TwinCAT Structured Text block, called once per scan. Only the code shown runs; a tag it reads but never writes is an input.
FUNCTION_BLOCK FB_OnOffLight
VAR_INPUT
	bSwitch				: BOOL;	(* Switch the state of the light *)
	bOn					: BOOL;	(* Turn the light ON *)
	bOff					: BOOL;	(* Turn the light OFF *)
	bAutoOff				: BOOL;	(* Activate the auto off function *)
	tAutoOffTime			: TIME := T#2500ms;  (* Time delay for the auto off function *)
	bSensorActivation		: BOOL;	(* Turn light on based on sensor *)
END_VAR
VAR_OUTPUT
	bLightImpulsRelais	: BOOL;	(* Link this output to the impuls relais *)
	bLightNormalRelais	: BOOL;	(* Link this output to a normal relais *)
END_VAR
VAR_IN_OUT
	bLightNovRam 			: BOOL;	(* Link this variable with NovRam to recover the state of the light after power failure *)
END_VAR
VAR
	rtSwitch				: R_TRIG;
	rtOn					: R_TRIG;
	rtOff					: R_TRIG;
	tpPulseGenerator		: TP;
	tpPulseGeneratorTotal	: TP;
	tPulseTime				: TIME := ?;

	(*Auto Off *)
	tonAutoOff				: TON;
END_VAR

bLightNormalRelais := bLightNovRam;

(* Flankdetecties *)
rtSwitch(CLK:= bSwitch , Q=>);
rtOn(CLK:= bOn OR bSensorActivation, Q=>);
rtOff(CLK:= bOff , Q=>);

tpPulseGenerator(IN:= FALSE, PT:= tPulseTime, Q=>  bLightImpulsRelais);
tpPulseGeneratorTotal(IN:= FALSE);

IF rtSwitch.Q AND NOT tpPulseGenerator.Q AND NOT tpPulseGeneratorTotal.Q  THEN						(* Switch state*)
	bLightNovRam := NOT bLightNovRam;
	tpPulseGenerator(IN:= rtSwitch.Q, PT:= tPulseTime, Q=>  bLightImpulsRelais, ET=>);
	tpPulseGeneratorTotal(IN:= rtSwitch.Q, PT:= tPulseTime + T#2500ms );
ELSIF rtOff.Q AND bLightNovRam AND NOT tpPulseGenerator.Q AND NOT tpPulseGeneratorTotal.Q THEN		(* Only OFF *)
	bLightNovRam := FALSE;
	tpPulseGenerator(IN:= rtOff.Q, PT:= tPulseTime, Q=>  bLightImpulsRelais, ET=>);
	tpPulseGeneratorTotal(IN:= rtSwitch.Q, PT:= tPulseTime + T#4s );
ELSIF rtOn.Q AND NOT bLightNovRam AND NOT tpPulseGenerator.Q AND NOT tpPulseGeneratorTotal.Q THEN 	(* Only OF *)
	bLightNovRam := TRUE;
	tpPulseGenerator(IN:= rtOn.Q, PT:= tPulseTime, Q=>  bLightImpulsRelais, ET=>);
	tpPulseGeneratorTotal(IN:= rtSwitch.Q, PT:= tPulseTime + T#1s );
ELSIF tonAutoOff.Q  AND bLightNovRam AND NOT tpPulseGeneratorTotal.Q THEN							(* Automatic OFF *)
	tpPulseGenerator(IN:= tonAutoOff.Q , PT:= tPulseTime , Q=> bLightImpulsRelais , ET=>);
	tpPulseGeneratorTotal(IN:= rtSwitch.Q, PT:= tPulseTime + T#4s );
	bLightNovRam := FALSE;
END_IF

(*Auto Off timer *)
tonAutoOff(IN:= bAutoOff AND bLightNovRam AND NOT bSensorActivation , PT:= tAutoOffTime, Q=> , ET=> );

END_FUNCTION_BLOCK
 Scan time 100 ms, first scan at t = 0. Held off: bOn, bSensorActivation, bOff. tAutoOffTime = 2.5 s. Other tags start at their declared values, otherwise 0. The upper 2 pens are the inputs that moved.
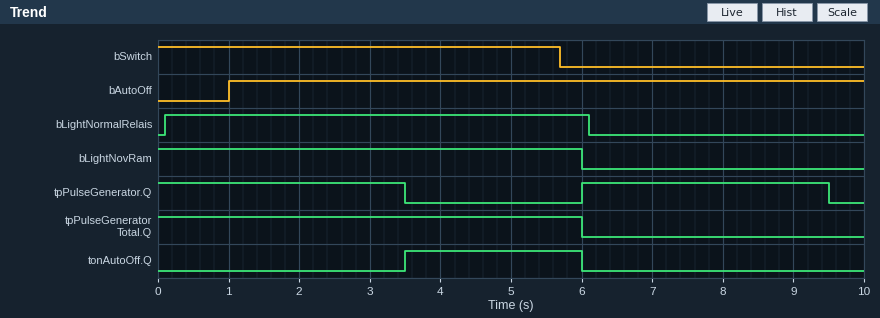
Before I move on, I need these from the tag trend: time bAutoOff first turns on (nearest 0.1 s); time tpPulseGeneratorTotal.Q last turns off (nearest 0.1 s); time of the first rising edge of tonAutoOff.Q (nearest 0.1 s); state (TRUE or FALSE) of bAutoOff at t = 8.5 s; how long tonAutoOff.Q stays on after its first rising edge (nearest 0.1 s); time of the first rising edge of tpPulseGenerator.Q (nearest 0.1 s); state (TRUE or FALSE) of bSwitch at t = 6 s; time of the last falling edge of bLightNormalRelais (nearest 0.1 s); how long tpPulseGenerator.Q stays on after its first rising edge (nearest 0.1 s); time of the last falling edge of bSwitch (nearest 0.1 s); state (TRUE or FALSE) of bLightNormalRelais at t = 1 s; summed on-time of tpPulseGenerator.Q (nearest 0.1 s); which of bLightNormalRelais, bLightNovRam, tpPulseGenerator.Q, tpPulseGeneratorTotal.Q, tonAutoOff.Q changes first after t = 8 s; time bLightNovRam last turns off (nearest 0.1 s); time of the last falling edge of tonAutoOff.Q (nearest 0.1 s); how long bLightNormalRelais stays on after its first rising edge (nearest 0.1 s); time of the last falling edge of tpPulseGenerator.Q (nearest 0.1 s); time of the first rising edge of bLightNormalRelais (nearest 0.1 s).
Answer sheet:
1.0 s
6.0 s
3.5 s
TRUE
2.5 s
6.0 s
FALSE
6.1 s
3.5 s
5.7 s
TRUE
7.0 s
tpPulseGenerator.Q
6.0 s
6.0 s
6.0 s
9.5 s
0.1 s
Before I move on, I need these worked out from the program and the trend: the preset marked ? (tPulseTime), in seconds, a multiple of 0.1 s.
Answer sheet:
3.5 s
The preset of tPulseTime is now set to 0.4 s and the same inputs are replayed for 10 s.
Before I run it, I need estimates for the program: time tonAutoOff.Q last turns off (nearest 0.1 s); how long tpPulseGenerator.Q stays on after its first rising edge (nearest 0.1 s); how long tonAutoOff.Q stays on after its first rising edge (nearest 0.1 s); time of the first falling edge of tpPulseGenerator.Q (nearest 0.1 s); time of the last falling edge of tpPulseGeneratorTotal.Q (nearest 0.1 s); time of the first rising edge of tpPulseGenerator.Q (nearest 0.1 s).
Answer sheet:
3.6 s
0.4 s
0.1 s
0.4 s
2.9 s
3.6 s
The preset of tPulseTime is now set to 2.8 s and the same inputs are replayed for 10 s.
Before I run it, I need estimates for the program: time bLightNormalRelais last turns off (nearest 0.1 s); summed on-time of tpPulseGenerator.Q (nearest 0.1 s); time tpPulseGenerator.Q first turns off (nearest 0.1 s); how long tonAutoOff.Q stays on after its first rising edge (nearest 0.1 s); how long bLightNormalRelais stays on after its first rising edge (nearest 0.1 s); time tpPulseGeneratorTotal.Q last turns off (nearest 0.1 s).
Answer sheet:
5.4 s
5.6 s
2.8 s
1.8 s
5.3 s
5.3 s
